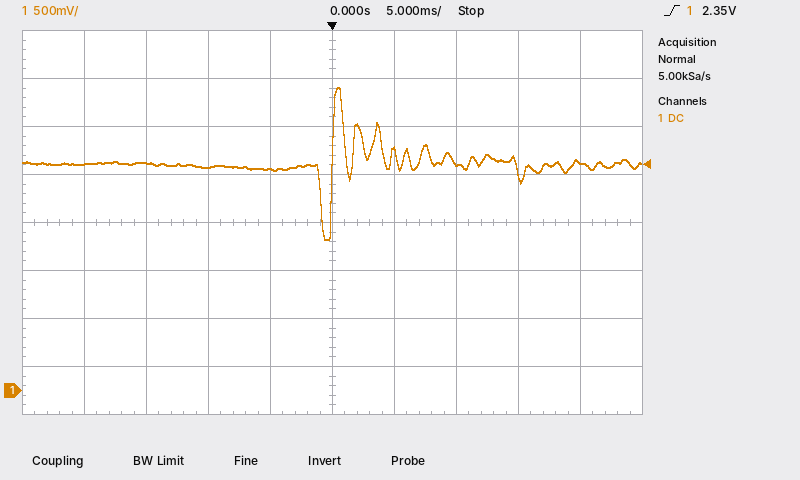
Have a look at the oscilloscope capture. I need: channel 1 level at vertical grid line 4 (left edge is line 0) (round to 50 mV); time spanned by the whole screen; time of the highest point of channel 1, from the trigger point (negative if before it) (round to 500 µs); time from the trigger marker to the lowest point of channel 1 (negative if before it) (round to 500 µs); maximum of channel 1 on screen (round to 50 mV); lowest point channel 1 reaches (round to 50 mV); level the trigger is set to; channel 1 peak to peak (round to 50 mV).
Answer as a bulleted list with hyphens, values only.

- 2.30 V
- 50 ms
- +500 µs
- -500 µs
- 3.15 V
- 1.55 V
- 2.35 V
- 1.60 V
